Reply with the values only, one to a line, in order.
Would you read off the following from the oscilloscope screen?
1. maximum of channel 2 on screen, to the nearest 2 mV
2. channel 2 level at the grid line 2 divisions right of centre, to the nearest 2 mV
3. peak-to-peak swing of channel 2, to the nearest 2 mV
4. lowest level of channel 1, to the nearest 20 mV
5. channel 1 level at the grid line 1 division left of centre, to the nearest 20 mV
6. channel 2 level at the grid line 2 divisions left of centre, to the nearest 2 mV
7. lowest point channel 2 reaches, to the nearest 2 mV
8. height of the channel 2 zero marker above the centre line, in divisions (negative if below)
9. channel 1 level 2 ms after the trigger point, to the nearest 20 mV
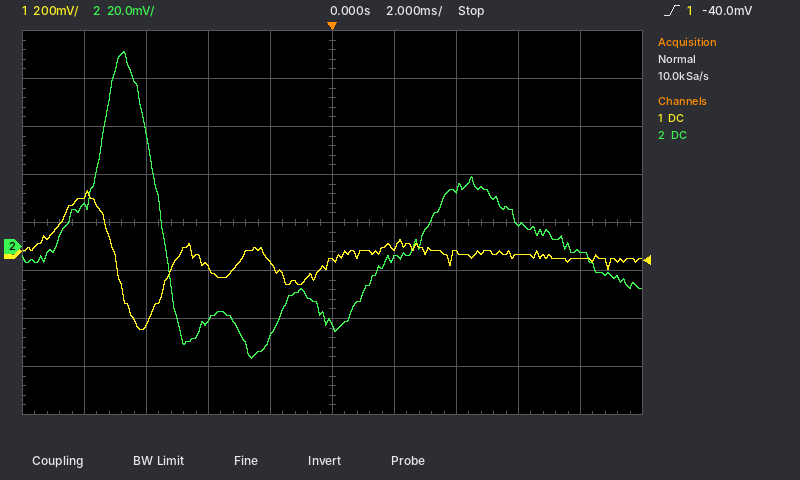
82 mV
24 mV
128 mV
-320 mV
-40 mV
-30 mV
-46 mV
-0.5 div
20 mV
